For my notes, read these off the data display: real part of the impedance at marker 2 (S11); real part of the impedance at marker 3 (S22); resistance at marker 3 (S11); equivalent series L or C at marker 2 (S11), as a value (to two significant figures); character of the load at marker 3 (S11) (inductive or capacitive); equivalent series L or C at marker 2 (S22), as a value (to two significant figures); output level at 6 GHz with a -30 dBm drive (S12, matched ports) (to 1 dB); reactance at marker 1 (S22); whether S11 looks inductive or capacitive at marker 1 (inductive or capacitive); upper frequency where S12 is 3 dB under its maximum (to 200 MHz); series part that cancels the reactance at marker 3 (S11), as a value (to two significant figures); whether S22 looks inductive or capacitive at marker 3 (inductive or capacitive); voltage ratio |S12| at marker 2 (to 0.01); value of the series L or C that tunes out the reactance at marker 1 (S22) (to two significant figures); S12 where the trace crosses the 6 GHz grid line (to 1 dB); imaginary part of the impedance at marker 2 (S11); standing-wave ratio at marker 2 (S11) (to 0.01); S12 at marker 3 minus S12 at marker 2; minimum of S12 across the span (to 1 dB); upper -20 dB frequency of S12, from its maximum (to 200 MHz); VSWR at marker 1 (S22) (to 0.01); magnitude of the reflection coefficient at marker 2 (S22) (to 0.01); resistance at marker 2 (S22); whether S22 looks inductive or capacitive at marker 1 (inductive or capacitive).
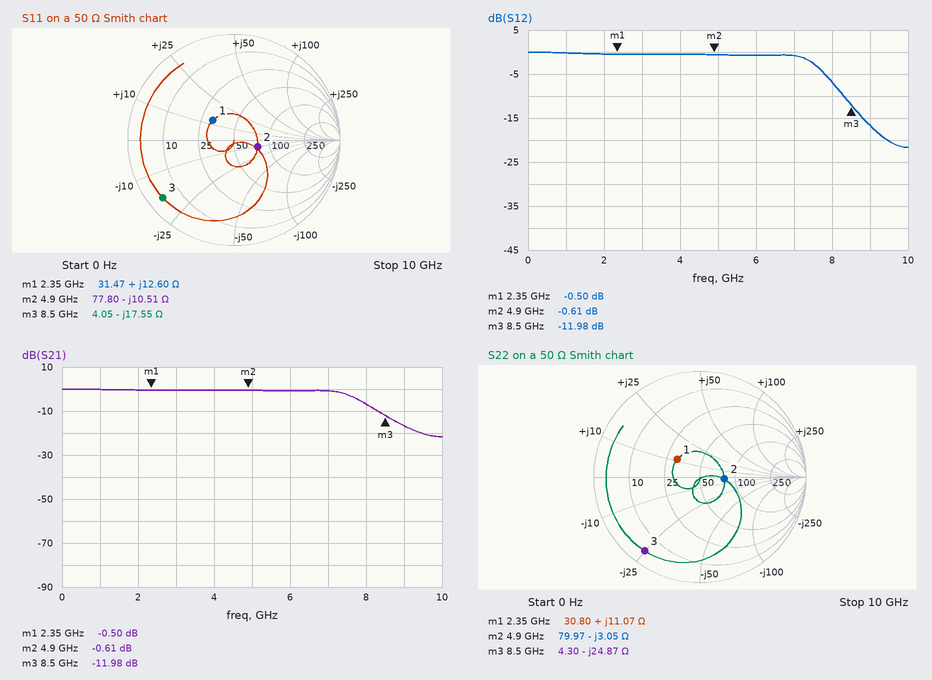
77.80 Ω
4.30 Ω
4.05 Ω
3.1 pF
capacitive
11 pF
-31 dBm
+11.07 Ω
inductive
7.6 GHz
330 pH
capacitive
0.93
6.1 pF
-1 dB
-10.51 Ω
1.60
-11.37 dB
-22 dB
9.4 GHz
1.75
0.23
79.97 Ω
inductive
